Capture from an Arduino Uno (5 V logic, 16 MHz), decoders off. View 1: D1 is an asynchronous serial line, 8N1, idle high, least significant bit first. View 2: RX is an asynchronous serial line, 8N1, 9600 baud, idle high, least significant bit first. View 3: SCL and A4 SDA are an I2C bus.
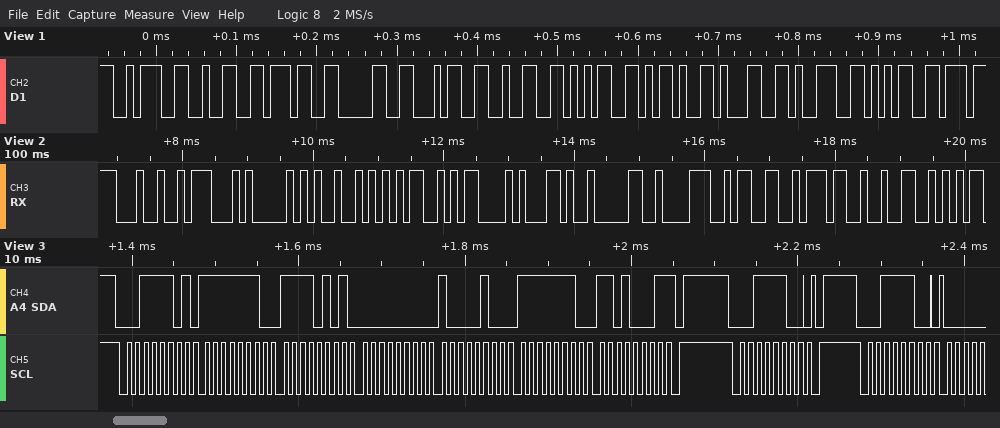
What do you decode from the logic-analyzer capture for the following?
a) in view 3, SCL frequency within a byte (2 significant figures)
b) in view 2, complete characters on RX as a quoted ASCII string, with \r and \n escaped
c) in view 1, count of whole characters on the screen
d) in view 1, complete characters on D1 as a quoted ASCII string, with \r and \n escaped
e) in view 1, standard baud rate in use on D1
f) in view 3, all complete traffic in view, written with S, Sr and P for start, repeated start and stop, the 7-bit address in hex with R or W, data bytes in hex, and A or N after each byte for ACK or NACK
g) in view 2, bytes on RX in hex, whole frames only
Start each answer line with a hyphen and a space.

- 100 kHz
- "$GPRMC,08372"
- 11
- ":270425-195"
- 115200 baud
- S 1ER A FE A F5 A 00 A 84 A FE A D1 N P S 1EW A P S 1EW A
- 0x24 0x47 0x50 0x52 0x4D 0x43 0x2C 0x30 0x38 0x33 0x37 0x32
